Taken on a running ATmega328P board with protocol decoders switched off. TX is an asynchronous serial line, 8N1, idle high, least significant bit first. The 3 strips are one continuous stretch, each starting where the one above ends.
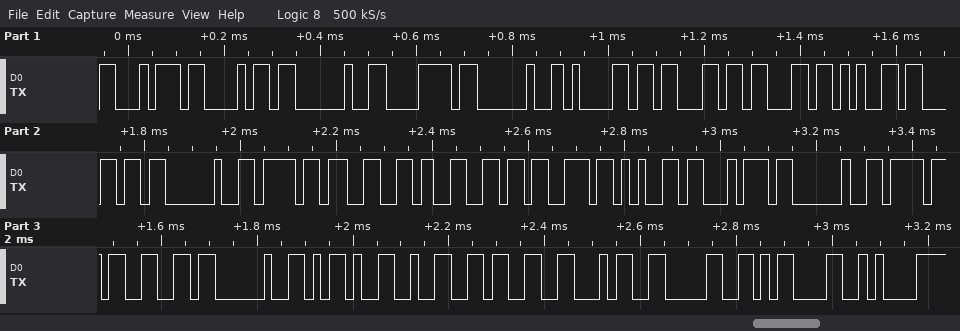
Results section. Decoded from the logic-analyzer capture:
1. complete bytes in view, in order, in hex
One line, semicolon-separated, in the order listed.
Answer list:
0x74 0x68 0x20 0x78 0x20 0x61 0x63 0x63 0x65 0x6C 0x20 0x6F 0x66 0x66 0x73 0x65 0x74 0x20 0x6F 0x66 0x20 0x2D 0x32 0x33 0x34 0x30 0x0D 0x0A
